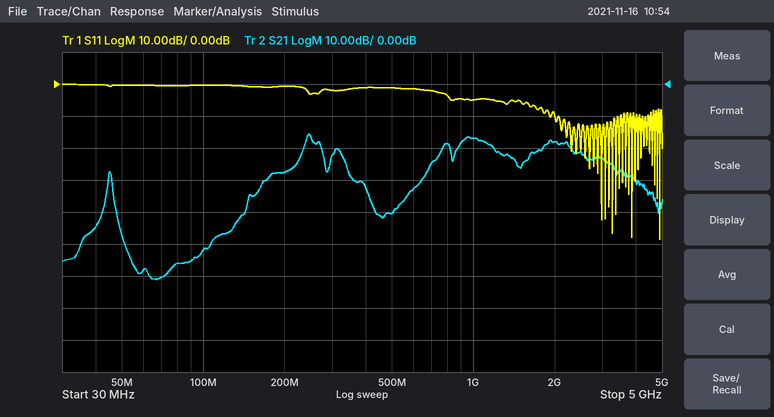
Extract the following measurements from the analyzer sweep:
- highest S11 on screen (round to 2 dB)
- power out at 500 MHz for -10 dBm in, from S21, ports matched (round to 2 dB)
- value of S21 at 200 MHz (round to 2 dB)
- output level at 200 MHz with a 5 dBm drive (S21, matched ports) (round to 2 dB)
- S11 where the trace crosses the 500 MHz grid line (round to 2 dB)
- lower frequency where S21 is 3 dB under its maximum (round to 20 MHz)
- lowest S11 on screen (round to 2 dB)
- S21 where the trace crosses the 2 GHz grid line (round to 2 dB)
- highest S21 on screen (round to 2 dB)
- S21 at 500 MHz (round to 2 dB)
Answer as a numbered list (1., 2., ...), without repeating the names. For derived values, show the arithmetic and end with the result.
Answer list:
1. 0 dB
2. -10 dBm + (-40 dB) = -50 dBm
3. -28 dB
4. 5 dBm + (-28 dB) = -22 dBm
5. -2 dB
6. 240 MHz
7. -48 dB
8. -18 dB
9. -16 dB
10. -40 dB
